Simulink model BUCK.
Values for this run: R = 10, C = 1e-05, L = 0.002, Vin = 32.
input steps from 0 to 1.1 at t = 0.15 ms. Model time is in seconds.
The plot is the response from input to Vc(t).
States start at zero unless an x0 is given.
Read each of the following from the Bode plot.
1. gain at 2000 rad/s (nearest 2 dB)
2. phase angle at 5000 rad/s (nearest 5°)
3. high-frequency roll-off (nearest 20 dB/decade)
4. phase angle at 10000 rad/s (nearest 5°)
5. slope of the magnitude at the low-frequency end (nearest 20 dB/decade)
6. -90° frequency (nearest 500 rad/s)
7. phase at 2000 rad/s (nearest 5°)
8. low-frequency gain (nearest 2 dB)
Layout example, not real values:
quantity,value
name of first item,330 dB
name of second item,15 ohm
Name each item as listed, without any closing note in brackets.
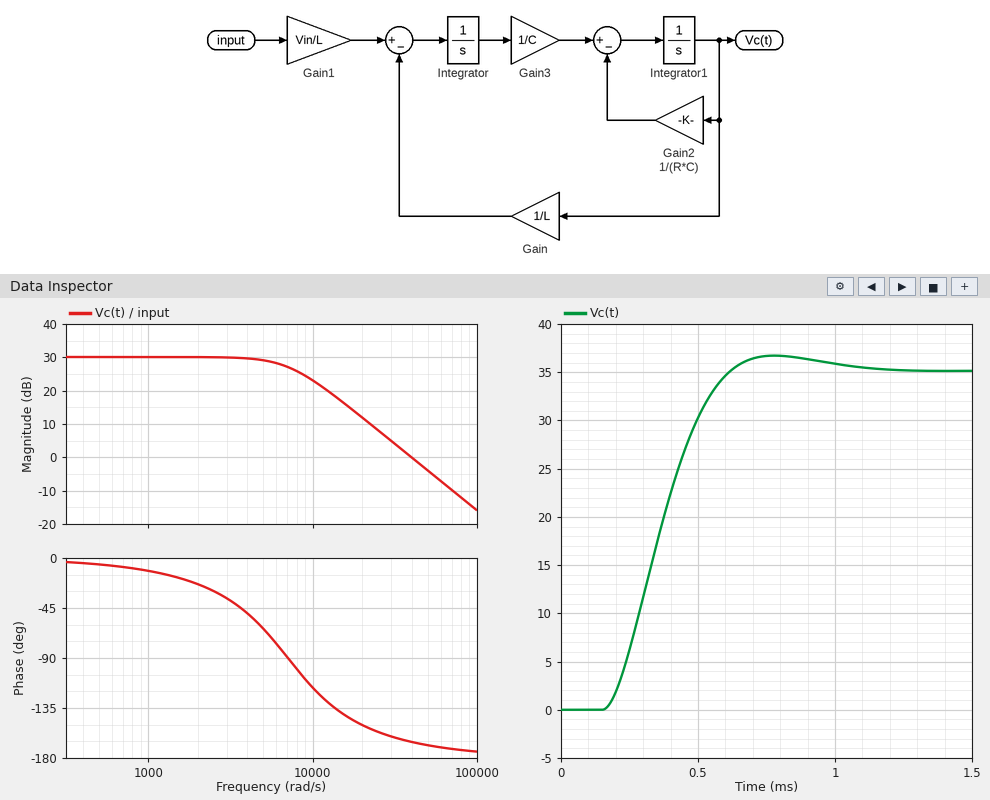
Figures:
quantity,value
gain at 2000 rad/s,30 dB
phase angle at 5000 rad/s,-65°
high-frequency roll-off,-40 dB/decade
phase angle at 10000 rad/s,-115°
slope of the magnitude at the low-frequency end,0 dB/decade
-90° frequency,7000 rad/s
phase at 2000 rad/s,-25°
low-frequency gain,30 dB
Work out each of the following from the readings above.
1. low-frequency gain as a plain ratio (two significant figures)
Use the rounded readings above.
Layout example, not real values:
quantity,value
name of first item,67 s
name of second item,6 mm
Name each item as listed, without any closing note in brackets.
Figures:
quantity,value
low-frequency gain as a plain ratio,32
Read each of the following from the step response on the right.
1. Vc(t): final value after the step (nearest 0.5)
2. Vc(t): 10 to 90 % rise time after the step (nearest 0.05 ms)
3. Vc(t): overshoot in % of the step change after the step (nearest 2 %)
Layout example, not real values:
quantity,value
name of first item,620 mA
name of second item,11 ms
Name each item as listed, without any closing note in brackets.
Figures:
quantity,value
Vc(t): final value after the step,35.0
Vc(t): 10 to 90 % rise time after the step,0.30 ms
Vc(t): overshoot in % of the step change after the step,4 %
